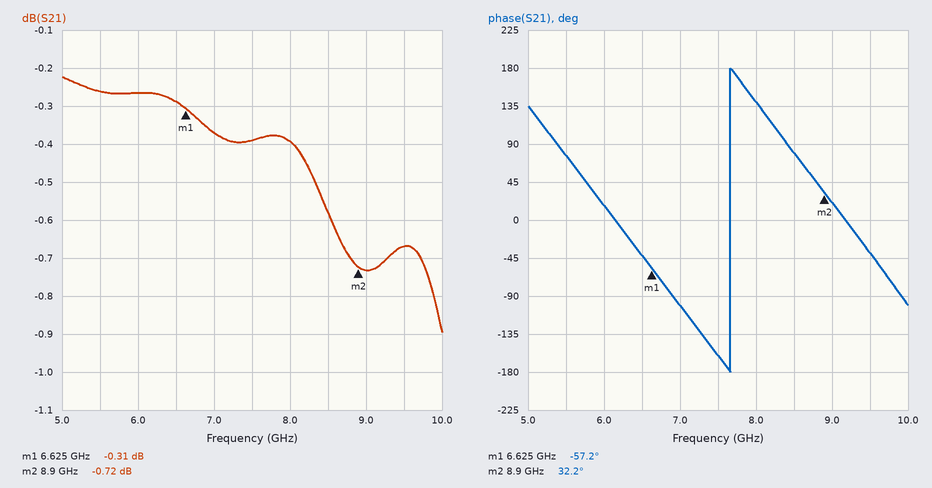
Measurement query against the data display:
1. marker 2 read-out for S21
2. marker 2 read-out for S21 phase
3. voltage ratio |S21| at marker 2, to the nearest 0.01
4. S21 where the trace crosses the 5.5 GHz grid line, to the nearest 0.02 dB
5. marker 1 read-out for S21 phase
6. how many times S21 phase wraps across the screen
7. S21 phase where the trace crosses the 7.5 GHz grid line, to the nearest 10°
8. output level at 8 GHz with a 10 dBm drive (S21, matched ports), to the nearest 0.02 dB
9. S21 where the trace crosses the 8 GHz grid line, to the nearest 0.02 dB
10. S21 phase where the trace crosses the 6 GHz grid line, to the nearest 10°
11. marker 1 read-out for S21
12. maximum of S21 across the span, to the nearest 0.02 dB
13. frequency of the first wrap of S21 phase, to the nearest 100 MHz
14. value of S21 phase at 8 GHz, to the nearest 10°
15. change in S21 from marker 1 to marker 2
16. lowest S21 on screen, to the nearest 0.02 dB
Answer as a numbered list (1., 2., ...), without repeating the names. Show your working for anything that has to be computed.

1. -0.72 dB
2. 32.2°
3. 10^(-0.72/20) ≈ 0.92
4. -0.26 dB
5. -57.2°
6. 1
7. -160°
8. 10 dBm + (-0.40 dB) = 9.60 dBm
9. -0.40 dB
10. 20°
11. -0.31 dB
12. -0.22 dB
13. 7.7 GHz
14. 140°
15. -0.72 − (-0.31) = -0.41 dB
16. -0.90 dB
